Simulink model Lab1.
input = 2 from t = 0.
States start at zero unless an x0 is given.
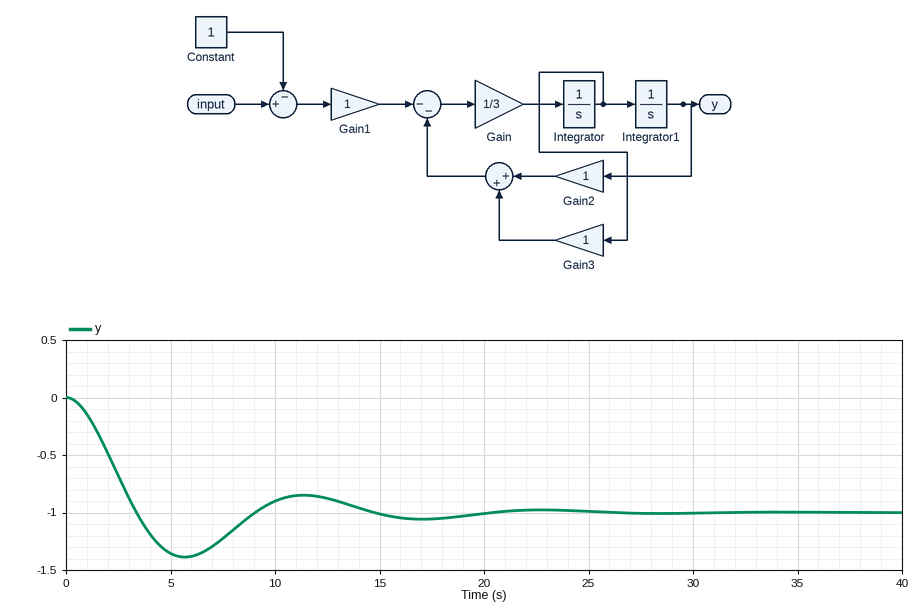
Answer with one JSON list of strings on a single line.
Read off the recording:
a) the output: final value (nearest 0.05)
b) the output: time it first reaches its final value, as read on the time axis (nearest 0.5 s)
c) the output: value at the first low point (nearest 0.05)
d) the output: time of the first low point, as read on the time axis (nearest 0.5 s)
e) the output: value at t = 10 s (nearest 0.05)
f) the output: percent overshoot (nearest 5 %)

["-1.00", "3.5 s", "-1.40", "5.5 s", "-0.90", "40 %"]
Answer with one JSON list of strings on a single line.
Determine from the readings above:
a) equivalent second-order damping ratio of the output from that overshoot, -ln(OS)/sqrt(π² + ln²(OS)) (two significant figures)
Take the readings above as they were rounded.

["0.28"]
